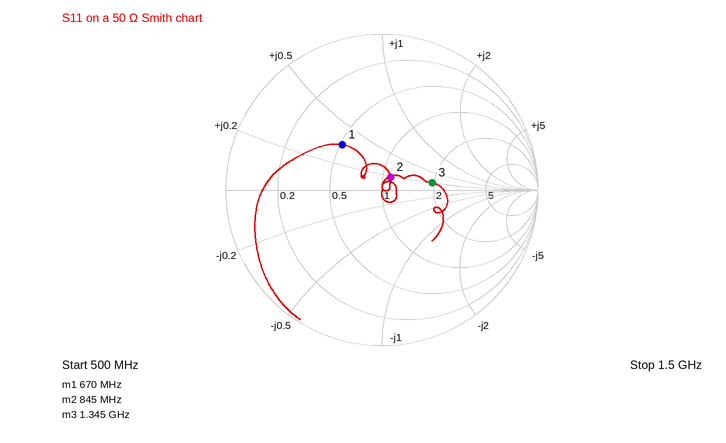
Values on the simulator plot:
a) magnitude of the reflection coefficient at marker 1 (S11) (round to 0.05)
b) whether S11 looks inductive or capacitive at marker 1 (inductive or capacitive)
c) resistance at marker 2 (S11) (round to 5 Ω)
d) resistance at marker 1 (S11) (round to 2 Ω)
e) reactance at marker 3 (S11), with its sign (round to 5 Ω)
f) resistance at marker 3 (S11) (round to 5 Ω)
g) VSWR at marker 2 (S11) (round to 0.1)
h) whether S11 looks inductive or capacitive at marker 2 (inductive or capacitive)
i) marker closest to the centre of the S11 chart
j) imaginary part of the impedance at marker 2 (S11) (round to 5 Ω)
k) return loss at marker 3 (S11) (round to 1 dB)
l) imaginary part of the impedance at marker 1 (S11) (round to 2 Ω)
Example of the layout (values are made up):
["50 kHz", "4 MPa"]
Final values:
["0.40", "inductive", "55 Ω", "26 Ω", "+10 Ω", "95 Ω", "1.2", "inductive", "marker 2", "+10 Ω", "10 dB", "+18 Ω"]
